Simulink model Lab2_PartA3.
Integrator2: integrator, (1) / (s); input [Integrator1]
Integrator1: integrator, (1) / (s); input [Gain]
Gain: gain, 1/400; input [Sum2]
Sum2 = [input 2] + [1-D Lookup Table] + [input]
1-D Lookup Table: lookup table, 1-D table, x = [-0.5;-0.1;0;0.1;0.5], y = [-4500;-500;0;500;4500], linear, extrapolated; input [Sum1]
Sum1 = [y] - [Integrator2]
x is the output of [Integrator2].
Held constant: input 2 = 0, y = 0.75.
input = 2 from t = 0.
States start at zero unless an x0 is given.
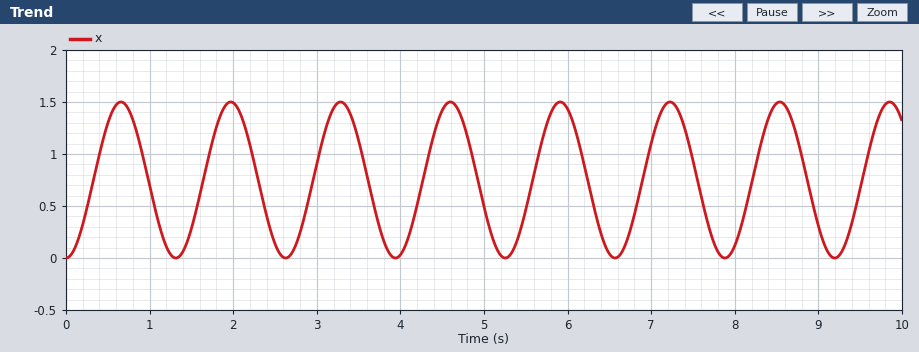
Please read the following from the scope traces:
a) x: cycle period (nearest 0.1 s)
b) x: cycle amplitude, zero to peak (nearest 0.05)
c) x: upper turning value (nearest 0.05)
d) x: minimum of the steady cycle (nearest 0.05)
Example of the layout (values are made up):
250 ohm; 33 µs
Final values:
1.3 s; 0.75; 1.50; 0.00
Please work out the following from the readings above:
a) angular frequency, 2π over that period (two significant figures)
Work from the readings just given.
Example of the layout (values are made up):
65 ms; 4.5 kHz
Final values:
4.8 rad/s
